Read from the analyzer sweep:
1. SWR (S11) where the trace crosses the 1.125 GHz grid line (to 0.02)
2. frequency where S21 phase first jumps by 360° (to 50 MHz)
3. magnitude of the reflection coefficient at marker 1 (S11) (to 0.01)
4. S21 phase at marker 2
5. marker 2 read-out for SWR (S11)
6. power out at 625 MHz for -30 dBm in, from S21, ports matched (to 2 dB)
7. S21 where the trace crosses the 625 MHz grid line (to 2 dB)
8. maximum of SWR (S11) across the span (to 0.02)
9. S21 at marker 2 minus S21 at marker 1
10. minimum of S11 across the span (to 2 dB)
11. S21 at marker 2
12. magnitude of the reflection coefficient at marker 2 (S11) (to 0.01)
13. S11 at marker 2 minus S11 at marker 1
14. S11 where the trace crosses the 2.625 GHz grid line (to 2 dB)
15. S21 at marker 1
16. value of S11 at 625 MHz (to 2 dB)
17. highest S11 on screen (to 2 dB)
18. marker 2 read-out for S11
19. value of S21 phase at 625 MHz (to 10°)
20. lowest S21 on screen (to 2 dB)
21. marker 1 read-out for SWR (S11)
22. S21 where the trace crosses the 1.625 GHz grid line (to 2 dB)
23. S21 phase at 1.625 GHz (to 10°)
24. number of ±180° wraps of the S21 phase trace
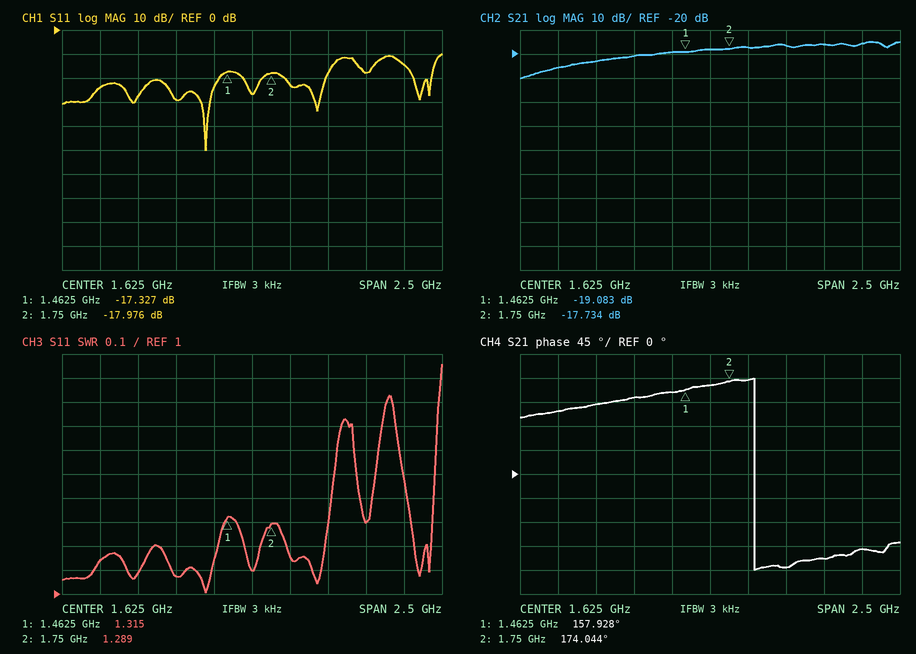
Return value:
1.08
1.90 GHz
0.14
174.044°
1.289
-56 dBm
-26 dB
1.96
1.349 dB
-50 dB
-17.734 dB
0.13
-0.649 dB
-14 dB
-19.083 dB
-24 dB
-10 dB
-17.976 dB
120°
-30 dB
1.315
-18 dB
170°
1
